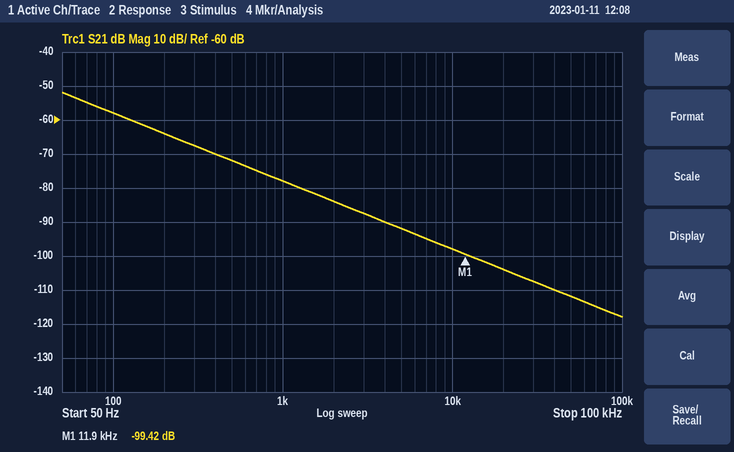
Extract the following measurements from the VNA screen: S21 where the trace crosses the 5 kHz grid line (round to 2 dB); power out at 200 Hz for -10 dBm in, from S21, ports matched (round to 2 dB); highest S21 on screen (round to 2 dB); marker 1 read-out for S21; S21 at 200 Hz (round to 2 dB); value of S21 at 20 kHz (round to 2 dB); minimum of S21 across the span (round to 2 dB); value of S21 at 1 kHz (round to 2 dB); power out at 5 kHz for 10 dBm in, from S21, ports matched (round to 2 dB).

-92 dB
-74 dBm
-52 dB
-99.42 dB
-64 dB
-104 dB
-118 dB
-78 dB
-82 dBm
